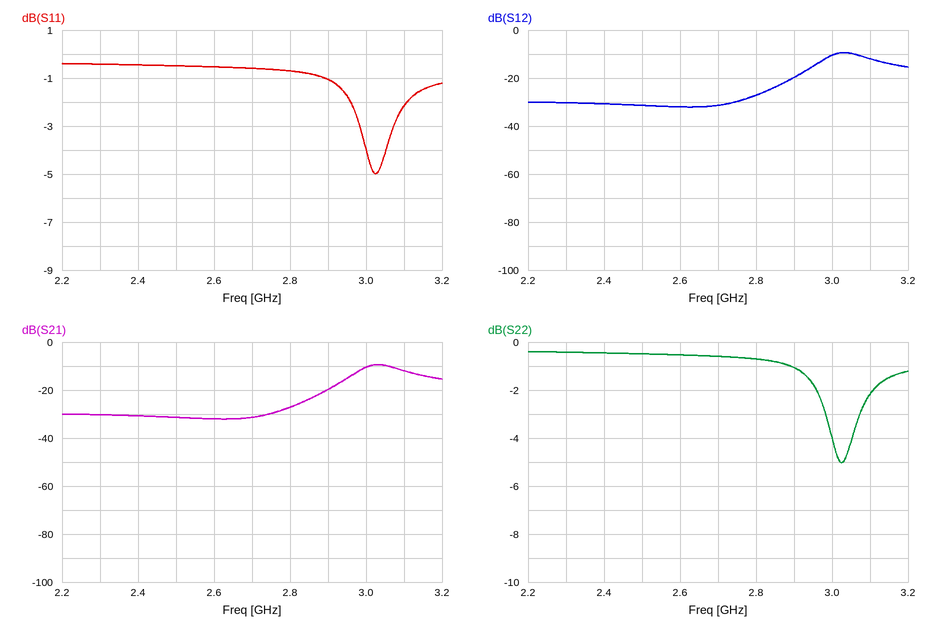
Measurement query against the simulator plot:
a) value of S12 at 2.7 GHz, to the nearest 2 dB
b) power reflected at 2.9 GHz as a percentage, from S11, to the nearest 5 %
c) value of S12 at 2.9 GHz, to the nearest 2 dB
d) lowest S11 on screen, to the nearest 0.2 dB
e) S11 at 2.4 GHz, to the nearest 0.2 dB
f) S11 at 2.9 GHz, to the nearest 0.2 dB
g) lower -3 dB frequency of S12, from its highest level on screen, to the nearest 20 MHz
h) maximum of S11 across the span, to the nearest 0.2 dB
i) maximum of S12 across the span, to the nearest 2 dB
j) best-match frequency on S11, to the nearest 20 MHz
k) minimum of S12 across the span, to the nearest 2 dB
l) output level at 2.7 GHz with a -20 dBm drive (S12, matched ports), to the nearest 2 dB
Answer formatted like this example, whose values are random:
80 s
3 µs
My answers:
-32 dB
80 %
-20 dB
-5.0 dB
-0.4 dB
-1.0 dB
2.98 GHz
-0.4 dB
-10 dB
3.02 GHz
-32 dB
-52 dBm
